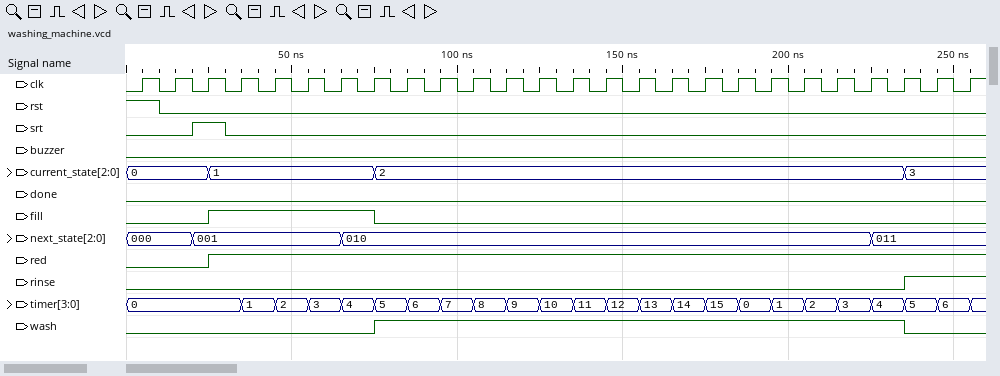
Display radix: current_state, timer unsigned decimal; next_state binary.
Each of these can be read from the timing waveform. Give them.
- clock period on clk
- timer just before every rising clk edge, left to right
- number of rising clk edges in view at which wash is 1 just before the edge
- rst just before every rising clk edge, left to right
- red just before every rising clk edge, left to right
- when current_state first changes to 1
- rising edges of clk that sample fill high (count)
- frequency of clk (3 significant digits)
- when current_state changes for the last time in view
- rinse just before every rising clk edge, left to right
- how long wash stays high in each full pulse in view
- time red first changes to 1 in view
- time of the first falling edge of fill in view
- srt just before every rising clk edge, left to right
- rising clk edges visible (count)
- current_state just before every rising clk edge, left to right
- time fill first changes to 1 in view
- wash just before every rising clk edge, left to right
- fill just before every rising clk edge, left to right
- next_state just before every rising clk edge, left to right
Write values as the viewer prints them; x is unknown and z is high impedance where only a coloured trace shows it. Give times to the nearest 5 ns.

10 ns
0, 0, 0, 0, 1, 2, 3, 4, 5, 6, 7, 8, 9, 10, 11, 12, 13, 14, 15, 0, 1, 2, 3, 4, 5, 6
16
1 0 0 0 0 0 0 0 0 0 0 0 0 0 0 0 0 0 0 0 0 0 0 0 0 0
0 0 0 1 1 1 1 1 1 1 1 1 1 1 1 1 1 1 1 1 1 1 1 1 1 1
25 ns
5
100 MHz
235 ns
0 0 0 0 0 0 0 0 0 0 0 0 0 0 0 0 0 0 0 0 0 0 0 0 1 1
160 ns
25 ns
75 ns
0 0 1 0 0 0 0 0 0 0 0 0 0 0 0 0 0 0 0 0 0 0 0 0 0 0
26
0, 0, 0, 1, 1, 1, 1, 1, 2, 2, 2, 2, 2, 2, 2, 2, 2, 2, 2, 2, 2, 2, 2, 2, 3, 3
25 ns
0 0 0 0 0 0 0 0 1 1 1 1 1 1 1 1 1 1 1 1 1 1 1 1 0 0
0 0 0 1 1 1 1 1 0 0 0 0 0 0 0 0 0 0 0 0 0 0 0 0 0 0
000, 000, 001, 001, 001, 001, 001, 010, 010, 010, 010, 010, 010, 010, 010, 010, 010, 010, 010, 010, 010, 010, 010, 011, 011, 011
